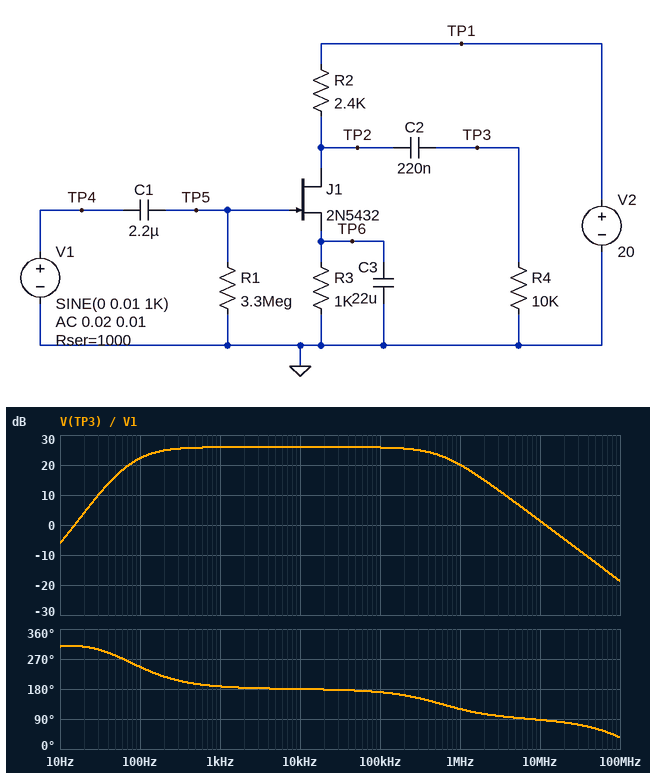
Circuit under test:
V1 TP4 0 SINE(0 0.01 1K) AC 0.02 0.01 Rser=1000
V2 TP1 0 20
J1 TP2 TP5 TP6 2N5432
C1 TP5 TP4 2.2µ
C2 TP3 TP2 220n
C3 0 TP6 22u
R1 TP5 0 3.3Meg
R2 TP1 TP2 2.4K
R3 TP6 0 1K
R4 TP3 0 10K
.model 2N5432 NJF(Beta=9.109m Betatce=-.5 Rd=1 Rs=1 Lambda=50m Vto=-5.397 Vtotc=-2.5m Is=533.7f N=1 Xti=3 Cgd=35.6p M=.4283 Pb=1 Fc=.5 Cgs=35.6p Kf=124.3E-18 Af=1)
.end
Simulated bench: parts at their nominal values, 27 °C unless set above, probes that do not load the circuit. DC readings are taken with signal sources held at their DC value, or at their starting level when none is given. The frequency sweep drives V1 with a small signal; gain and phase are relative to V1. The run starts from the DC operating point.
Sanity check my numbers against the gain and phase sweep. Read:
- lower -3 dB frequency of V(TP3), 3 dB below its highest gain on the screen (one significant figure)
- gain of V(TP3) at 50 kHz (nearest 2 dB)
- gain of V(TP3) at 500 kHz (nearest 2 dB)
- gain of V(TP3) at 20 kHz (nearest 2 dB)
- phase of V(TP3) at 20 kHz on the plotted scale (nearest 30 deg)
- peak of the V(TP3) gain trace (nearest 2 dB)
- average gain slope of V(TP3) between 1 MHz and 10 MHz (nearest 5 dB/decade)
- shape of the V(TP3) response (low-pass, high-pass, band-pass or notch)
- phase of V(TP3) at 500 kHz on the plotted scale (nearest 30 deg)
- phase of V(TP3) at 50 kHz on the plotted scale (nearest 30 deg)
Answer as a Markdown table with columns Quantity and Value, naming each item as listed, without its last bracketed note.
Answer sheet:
| Quantity | Value |
|---|---|
| lower -3 dB frequency of V(TP3), 3 dB below its highest gain on the screen | 100 Hz |
| gain of V(TP3) at 50 kHz | 26 dB |
| gain of V(TP3) at 500 kHz | 24 dB |
| gain of V(TP3) at 20 kHz | 26 dB |
| phase of V(TP3) at 20 kHz on the plotted scale | 180 deg |
| peak of the V(TP3) gain trace | 26 dB |
| average gain slope of V(TP3) between 1 MHz and 10 MHz | -20 dB/decade |
| shape of the V(TP3) response | band-pass |
| phase of V(TP3) at 500 kHz on the plotted scale | 150 deg |
| phase of V(TP3) at 50 kHz on the plotted scale | 180 deg |
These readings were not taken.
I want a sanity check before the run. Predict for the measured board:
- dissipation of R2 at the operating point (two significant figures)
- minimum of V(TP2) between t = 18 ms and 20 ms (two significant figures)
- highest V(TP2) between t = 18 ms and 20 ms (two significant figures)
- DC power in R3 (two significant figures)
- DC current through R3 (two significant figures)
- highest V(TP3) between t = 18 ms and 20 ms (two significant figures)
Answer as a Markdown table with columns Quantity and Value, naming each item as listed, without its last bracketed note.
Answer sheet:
| Quantity | Value |
|---|---|
| dissipation of R2 at the operating point | 54 mW |
| minimum of V(TP2) between t = 18 ms and 20 ms | 8.4 V |
| highest V(TP2) between t = 18 ms and 20 ms | 8.8 V |
| DC power in R3 | 22 mW |
| DC current through R3 | 4.7 mA |
| highest V(TP3) between t = 18 ms and 20 ms | 200 mV |
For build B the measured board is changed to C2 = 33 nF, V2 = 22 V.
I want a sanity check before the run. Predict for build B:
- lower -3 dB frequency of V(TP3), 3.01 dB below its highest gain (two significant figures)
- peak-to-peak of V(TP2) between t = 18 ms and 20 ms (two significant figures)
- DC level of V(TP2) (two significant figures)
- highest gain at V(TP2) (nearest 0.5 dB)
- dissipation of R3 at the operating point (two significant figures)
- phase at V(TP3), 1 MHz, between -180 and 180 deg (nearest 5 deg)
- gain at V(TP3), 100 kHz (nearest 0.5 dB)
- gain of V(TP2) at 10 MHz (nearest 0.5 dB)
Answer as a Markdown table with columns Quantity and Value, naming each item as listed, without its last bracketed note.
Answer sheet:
| Quantity | Value |
|---|---|
| lower -3 dB frequency of V(TP3), 3.01 dB below its highest gain | 430 Hz |
| peak-to-peak of V(TP2) between t = 18 ms and 20 ms | 430 mV |
| DC level of V(TP2) | 11 V |
| highest gain at V(TP2) | 27.0 dB |
| dissipation of R3 at the operating point | 23 mW |
| phase at V(TP3), 1 MHz, between -180 and 180 deg | 120 deg |
| gain at V(TP3), 100 kHz | 26.5 dB |
| gain of V(TP2) at 10 MHz | 2.0 dB |
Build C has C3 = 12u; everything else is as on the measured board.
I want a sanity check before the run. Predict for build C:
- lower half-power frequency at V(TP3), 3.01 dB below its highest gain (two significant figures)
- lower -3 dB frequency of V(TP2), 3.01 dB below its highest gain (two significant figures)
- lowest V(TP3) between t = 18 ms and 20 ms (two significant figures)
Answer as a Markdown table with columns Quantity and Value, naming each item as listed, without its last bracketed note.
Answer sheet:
| Quantity | Value |
|---|---|
| lower half-power frequency at V(TP3), 3.01 dB below its highest gain | 170 Hz |
| lower -3 dB frequency of V(TP2), 3.01 dB below its highest gain | 140 Hz |
| lowest V(TP3) between t = 18 ms and 20 ms | -200 mV |
